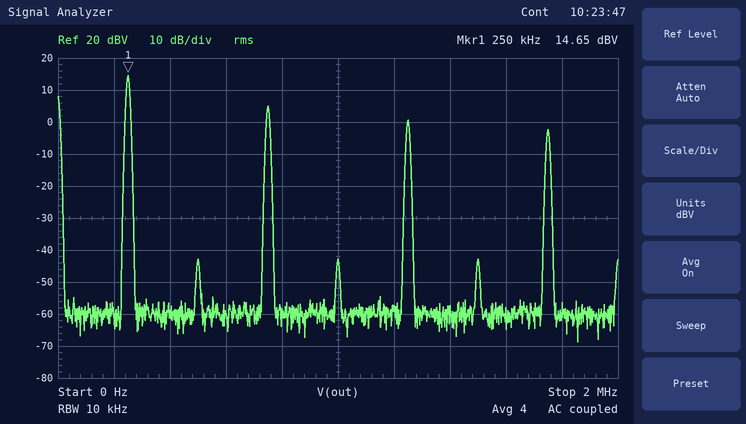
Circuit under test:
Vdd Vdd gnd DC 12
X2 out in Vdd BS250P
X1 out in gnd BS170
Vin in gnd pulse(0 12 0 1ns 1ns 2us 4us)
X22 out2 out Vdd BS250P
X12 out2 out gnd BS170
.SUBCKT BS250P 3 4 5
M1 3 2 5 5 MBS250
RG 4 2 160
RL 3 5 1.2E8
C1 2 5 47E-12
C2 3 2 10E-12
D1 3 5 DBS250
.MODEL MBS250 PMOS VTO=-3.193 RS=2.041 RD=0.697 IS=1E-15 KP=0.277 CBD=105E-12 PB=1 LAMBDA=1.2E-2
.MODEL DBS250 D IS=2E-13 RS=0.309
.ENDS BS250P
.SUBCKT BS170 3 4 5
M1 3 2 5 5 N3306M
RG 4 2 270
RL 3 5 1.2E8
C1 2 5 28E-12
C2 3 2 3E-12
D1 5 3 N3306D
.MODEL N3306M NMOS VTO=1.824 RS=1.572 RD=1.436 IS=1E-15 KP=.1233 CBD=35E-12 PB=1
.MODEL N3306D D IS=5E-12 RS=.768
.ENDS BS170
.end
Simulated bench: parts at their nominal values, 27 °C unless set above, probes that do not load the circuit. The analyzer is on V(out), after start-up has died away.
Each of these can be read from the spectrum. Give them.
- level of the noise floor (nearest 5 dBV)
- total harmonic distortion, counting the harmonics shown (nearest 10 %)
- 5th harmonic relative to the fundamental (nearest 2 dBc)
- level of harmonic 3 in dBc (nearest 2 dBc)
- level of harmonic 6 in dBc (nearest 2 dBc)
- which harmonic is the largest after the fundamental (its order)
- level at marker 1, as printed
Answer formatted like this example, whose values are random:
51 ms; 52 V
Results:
-60 dBV; 40 %; -14 dBc; -10 dBc; -58 dBc; 3; 14.65 dBV
